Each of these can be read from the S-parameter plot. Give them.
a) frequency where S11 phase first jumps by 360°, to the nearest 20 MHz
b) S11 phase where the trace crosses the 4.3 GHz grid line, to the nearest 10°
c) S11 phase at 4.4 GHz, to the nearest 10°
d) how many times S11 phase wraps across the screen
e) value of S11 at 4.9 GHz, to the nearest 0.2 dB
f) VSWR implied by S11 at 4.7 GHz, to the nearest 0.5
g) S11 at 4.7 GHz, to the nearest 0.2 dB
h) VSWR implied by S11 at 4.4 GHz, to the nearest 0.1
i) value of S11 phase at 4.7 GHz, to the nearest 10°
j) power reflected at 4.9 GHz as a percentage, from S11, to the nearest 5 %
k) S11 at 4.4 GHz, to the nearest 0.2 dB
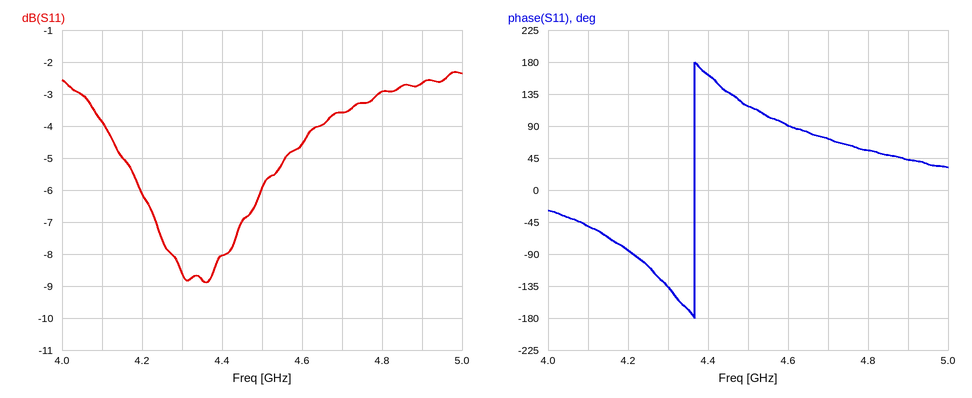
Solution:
4.36 GHz
-140°
160°
1
-2.6 dB
5.0
-3.6 dB
2.3
70°
55 %
-8.0 dB
